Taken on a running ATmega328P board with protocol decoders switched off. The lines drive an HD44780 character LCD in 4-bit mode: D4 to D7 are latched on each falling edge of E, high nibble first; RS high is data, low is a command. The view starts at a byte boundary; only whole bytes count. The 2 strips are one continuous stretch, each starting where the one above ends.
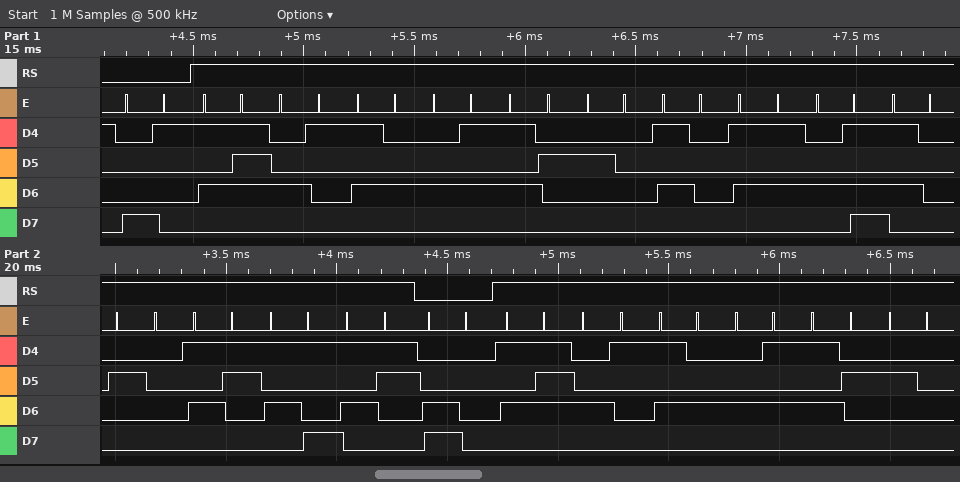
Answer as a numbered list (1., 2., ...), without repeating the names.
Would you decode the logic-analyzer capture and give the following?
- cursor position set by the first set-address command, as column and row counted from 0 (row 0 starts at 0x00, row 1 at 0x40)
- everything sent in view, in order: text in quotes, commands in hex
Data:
1. column 1, row 0
2. 0x81 "WATER PUMP SYS" 0xC0 "WATER "
